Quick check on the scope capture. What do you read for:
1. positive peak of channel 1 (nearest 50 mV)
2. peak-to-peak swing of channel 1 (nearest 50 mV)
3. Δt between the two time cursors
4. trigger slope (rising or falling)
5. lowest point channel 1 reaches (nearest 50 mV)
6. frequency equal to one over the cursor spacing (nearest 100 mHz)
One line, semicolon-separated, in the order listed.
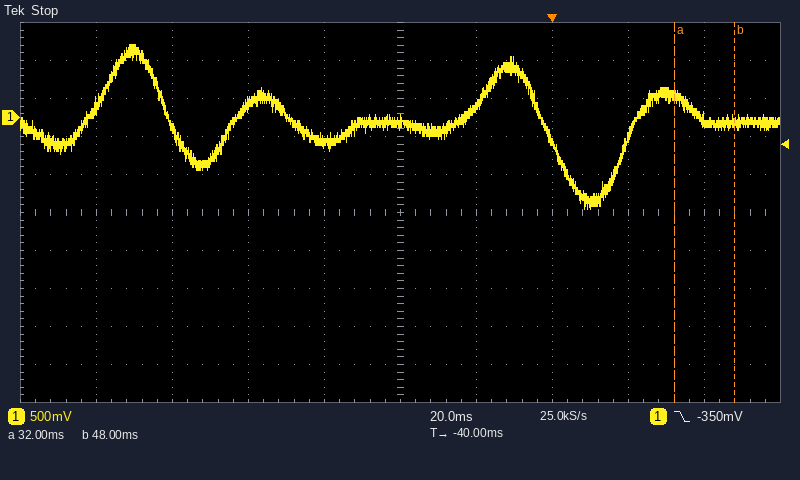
950 mV; 2.15 V; 16 ms; falling; -1.20 V; 62.5 Hz
